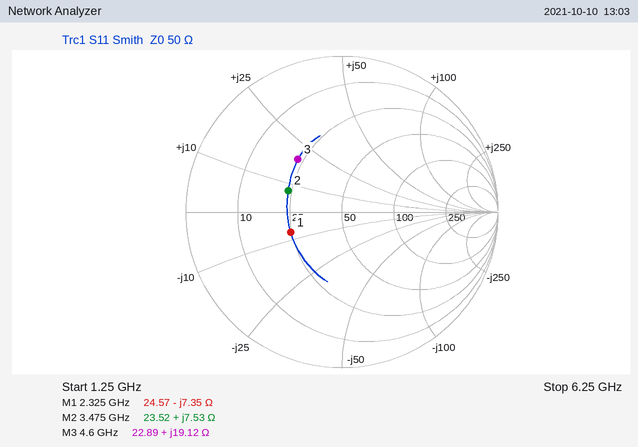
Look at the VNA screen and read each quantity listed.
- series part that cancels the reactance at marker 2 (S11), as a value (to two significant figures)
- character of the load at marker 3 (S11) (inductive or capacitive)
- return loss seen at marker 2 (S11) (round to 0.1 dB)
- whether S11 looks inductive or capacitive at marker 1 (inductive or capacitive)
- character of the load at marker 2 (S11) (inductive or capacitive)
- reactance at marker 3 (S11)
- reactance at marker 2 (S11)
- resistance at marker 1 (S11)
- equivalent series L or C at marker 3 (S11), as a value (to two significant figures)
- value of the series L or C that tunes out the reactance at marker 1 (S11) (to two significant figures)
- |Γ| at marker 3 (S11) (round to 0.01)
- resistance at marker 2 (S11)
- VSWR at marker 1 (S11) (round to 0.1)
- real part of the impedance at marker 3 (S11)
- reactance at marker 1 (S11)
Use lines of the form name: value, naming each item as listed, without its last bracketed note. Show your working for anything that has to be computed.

series part that cancels the reactance at marker 2 (S11), as a value: C = 1/(2π × 3.475 GHz × 7.53 Ω) ≈ 6.1 pF
character of the load at marker 3 (S11): inductive
return loss seen at marker 2 (S11): 8.6 dB
whether S11 looks inductive or capacitive at marker 1: capacitive
character of the load at marker 2 (S11): inductive
reactance at marker 3: +19.12 Ω
reactance at marker 2: +7.53 Ω
resistance at marker 1: 24.57 Ω
equivalent series L or C at marker 3 (S11), as a value: L = 19.12 Ω/(2π × 4.6 GHz) ≈ 662 pH, so 660 pH to two significant figures
value of the series L or C that tunes out the reactance at marker 1 (S11): L = 7.35 Ω/(2π × 2.325 GHz) ≈ 503 pH, so 500 pH to two significant figures
|Γ| at marker 3 (S11): 0.44
resistance at marker 2: 23.52 Ω
VSWR at marker 1 (S11): 2.1
real part of the impedance at marker 3: 22.89 Ω
reactance at marker 1: -7.35 Ω
